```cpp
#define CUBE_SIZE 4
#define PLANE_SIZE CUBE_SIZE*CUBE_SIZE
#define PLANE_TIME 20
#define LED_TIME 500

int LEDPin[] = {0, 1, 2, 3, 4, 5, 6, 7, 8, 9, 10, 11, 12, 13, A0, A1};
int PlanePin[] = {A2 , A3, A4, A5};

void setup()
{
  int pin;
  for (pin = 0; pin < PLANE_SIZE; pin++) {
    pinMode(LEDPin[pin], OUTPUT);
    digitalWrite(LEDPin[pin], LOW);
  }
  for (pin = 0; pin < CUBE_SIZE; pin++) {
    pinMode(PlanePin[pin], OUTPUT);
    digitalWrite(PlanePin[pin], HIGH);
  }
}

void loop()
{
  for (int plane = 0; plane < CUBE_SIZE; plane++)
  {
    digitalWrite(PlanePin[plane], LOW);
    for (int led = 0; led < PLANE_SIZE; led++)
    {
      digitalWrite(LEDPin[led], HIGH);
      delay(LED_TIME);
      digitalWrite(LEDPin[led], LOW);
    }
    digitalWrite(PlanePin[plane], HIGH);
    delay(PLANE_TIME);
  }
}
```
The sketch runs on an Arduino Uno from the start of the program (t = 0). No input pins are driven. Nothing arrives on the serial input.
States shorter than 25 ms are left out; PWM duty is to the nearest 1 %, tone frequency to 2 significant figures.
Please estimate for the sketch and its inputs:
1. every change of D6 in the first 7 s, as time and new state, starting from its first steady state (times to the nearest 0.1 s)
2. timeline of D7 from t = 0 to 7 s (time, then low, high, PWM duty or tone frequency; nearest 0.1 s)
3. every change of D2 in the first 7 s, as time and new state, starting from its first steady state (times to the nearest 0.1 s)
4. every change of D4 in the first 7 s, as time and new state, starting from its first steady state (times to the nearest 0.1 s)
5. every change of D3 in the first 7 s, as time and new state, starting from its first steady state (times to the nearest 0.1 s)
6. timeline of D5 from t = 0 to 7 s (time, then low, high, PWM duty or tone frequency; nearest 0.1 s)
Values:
0 s low; 3 s high; 3.5 s low
0 s low; 3.5 s high; 4 s low
0 s low; 1 s high; 1.5 s low
0 s low; 2 s high; 2.5 s low
0 s low; 1.5 s high; 2 s low
0 s low; 2.5 s high; 3 s low
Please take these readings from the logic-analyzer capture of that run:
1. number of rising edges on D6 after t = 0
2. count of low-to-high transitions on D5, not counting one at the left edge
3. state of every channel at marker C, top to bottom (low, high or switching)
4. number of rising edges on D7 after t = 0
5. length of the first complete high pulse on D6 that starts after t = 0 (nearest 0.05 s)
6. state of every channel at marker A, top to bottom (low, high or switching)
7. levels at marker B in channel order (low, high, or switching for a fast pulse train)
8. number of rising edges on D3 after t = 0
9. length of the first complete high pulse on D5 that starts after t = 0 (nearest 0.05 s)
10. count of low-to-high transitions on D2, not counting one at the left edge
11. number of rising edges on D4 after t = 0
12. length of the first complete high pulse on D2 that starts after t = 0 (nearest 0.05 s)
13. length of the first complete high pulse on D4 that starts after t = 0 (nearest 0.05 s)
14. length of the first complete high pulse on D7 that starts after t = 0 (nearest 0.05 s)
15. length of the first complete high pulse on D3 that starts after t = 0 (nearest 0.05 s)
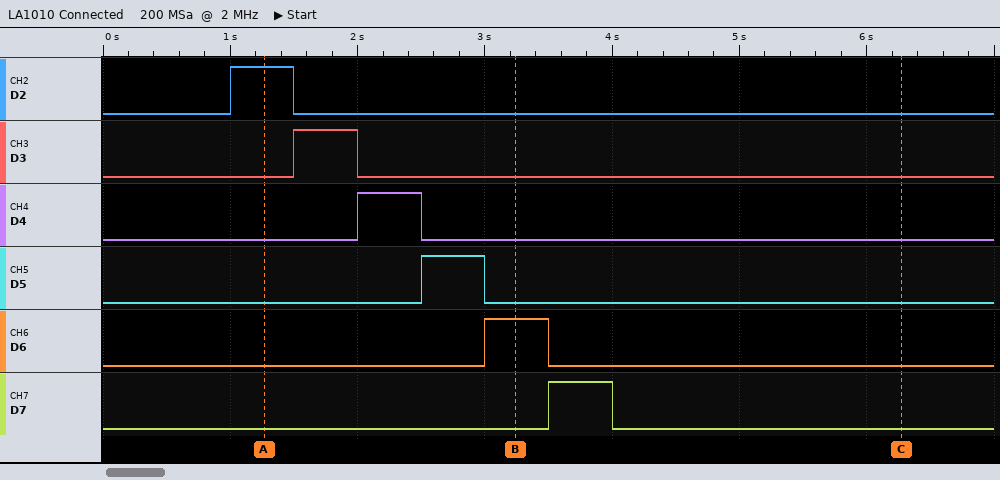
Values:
1
1
D2 low, D3 low, D4 low, D5 low, D6 low, D7 low
1
0.50 s
D2 high, D3 low, D4 low, D5 low, D6 low, D7 low
D2 low, D3 low, D4 low, D5 low, D6 high, D7 low
1
0.50 s
1
1
0.50 s
0.50 s
0.50 s
0.50 s
